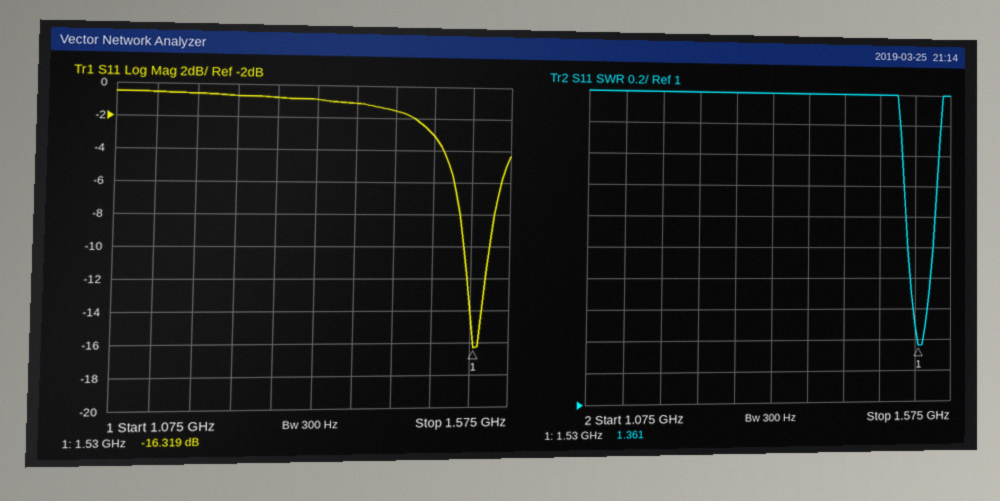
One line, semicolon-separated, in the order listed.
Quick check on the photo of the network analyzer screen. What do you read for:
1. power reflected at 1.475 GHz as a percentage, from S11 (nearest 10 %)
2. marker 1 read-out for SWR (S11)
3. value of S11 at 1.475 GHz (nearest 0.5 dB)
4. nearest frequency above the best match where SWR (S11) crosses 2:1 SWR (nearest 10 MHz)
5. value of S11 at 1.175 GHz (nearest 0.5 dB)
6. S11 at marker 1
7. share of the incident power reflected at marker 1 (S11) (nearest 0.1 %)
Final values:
50 %; 1.361; -3.0 dB; 1.55 GHz; -0.5 dB; -16.319 dB; 2.3 %
